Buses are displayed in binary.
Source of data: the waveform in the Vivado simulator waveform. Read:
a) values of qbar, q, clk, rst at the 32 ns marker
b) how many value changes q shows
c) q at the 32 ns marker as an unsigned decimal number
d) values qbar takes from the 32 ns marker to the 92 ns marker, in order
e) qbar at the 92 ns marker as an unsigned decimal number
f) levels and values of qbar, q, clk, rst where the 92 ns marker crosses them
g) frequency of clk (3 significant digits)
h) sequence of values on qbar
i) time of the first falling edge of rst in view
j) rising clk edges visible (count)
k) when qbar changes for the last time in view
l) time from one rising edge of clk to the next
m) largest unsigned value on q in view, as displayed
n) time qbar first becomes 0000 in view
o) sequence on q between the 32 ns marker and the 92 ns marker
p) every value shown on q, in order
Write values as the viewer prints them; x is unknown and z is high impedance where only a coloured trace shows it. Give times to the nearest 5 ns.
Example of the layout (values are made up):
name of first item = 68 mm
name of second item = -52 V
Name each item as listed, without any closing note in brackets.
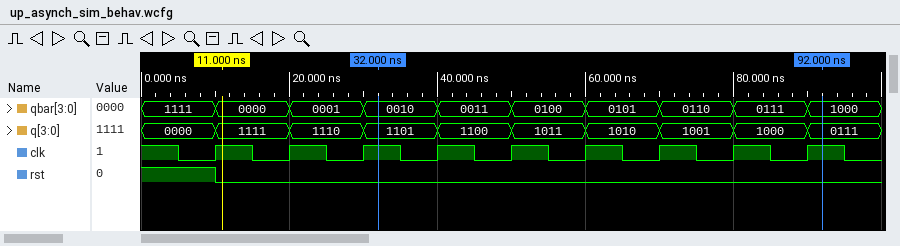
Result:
values of qbar, q, clk, rst at the 32 ns marker = qbar=0010, q=1101, clk=1, rst=0
how many value changes q shows = 9
q at the 32 ns marker as an unsigned decimal number = 13
values qbar takes from the 32 ns marker to the 92 ns marker, in order = 0010, 0011, 0100, 0101, 0110, 0111, 1000
qbar at the 92 ns marker as an unsigned decimal number = 8
levels and values of qbar, q, clk, rst where the 92 ns marker crosses them = qbar=1000, q=0111, clk=1, rst=0
frequency of clk = 100 MHz
sequence of values on qbar = 1111, 0000, 0001, 0010, 0011, 0100, 0101, 0110, 0111, 1000
time of the first falling edge of rst in view = 10 ns
rising clk edges visible = 9
when qbar changes for the last time in view = 90 ns
time from one rising edge of clk to the next = 10 ns
largest unsigned value on q in view, as displayed = 1111
time qbar first becomes 0000 in view = 10 ns
sequence on q between the 32 ns marker and the 92 ns marker = 1101, 1100, 1011, 1010, 1001, 1000, 0111
every value shown on q, in order = 0000, 1111, 1110, 1101, 1100, 1011, 1010, 1001, 1000, 0111
